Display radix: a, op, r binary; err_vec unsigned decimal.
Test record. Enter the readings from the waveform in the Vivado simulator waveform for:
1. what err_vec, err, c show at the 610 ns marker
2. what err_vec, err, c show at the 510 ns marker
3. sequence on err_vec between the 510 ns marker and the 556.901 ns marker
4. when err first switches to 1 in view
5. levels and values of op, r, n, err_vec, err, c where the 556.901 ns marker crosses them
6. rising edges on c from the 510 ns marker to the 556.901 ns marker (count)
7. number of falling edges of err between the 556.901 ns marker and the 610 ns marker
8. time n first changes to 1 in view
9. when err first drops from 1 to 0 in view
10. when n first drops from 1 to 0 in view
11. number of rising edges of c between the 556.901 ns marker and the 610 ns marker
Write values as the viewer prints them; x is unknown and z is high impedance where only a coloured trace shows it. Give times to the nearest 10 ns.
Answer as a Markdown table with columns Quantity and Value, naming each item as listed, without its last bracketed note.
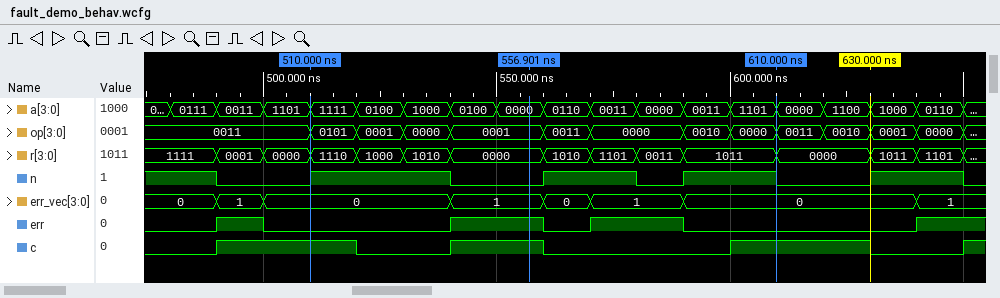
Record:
| Quantity | Value |
|---|---|
| what err_vec, err, c show at the 610 ns marker | err_vec=0, err=0, c=1 |
| what err_vec, err, c show at the 510 ns marker | err_vec=0, err=0, c=1 |
| sequence on err_vec between the 510 ns marker and the 556.901 ns marker | 0, 1 |
| when err first switches to 1 in view | 490 ns |
| levels and values of op, r, n, err_vec, err, c where the 556.901 ns marker crosses them | op=0001, r=0000, n=0, err_vec=1, err=1, c=1 |
| rising edges on c from the 510 ns marker to the 556.901 ns marker | 1 |
| number of falling edges of err between the 556.901 ns marker and the 610 ns marker | 2 |
| time n first changes to 1 in view | 510 ns |
| when err first drops from 1 to 0 in view | 500 ns |
| when n first drops from 1 to 0 in view | 490 ns |
| number of rising edges of c between the 556.901 ns marker and the 610 ns marker | 1 |
